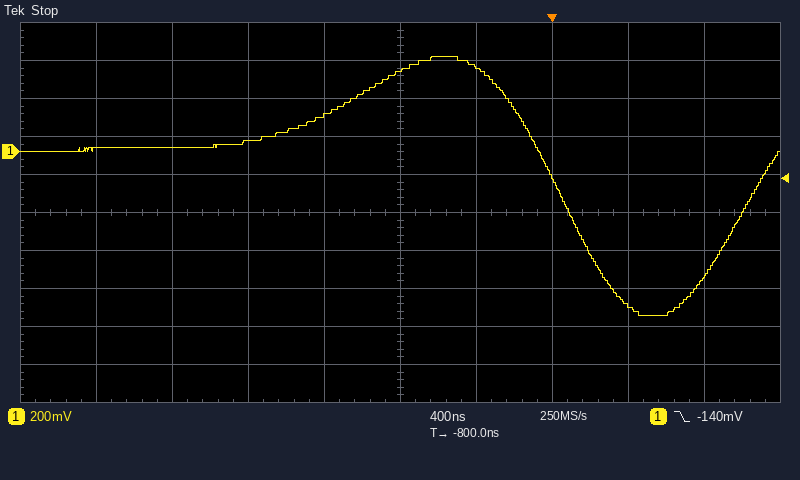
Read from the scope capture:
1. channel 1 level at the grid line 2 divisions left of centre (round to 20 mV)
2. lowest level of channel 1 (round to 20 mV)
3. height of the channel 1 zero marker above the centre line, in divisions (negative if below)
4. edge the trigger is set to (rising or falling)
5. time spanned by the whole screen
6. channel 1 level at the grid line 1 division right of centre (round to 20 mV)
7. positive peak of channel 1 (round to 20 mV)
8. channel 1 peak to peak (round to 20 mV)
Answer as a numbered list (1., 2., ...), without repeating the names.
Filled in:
1. 60 mV
2. -860 mV
3. +1.6 div
4. falling
5. 4 µs
6. 440 mV
7. 500 mV
8. 1.36 V
